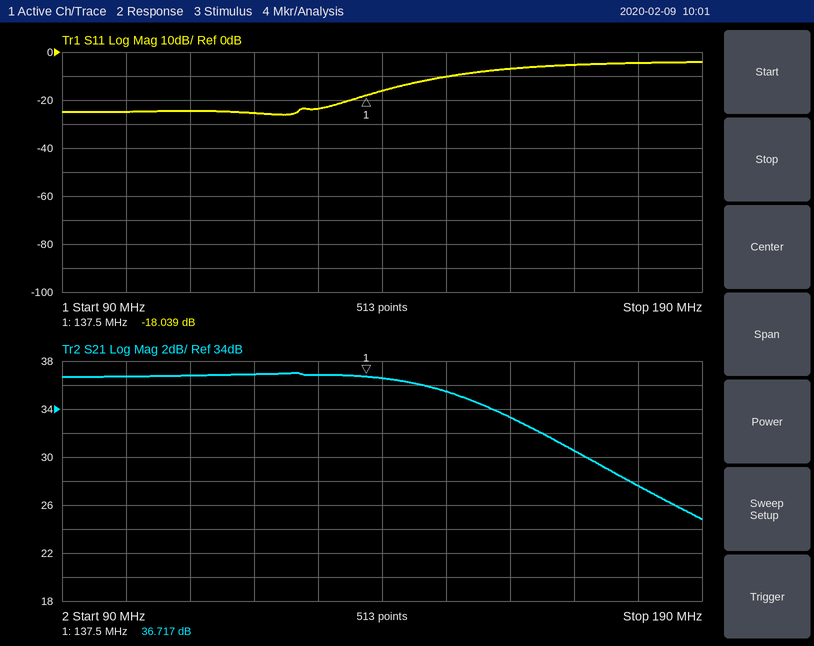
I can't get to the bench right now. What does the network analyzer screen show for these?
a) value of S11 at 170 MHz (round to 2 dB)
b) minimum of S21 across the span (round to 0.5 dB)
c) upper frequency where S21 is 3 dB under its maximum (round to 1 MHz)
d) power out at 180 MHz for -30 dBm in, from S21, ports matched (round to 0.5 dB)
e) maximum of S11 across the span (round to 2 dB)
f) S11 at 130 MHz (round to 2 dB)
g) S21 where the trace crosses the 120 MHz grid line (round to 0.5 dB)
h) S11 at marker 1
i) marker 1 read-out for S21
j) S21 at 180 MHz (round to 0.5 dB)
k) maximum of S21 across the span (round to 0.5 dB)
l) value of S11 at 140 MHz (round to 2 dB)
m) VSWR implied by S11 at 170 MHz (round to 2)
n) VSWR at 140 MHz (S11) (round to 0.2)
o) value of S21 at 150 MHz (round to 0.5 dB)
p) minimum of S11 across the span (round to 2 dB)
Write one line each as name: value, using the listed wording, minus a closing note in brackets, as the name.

value of S11 at 170 MHz: -6 dB
minimum of S21 across the span: 25.0 dB
upper frequency where S21 is 3 dB under its maximum: 157 MHz
power out at 180 MHz for -30 dBm in, from S21, ports matched: -2.5 dBm
maximum of S11 across the span: -4 dB
S11 at 130 MHz: -24 dB
S21 where the trace crosses the 120 MHz grid line: 37.0 dB
S11 at marker 1: -18.039 dB
marker 1 read-out for S21: 36.717 dB
S21 at 180 MHz: 27.5 dB
maximum of S21 across the span: 37.0 dB
value of S11 at 140 MHz: -16 dB
VSWR implied by S11 at 170 MHz: 4
VSWR at 140 MHz (S11): 1.4
value of S21 at 150 MHz: 35.5 dB
minimum of S11 across the span: -26 dB
